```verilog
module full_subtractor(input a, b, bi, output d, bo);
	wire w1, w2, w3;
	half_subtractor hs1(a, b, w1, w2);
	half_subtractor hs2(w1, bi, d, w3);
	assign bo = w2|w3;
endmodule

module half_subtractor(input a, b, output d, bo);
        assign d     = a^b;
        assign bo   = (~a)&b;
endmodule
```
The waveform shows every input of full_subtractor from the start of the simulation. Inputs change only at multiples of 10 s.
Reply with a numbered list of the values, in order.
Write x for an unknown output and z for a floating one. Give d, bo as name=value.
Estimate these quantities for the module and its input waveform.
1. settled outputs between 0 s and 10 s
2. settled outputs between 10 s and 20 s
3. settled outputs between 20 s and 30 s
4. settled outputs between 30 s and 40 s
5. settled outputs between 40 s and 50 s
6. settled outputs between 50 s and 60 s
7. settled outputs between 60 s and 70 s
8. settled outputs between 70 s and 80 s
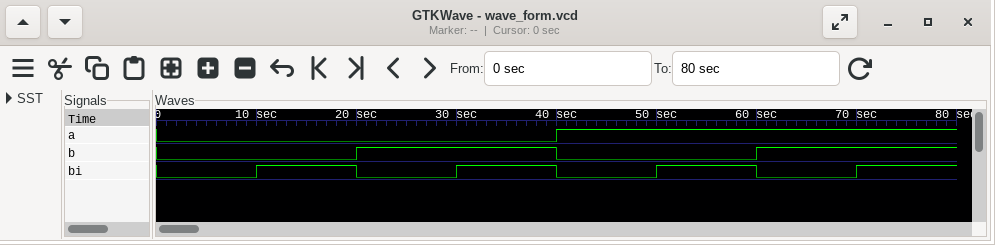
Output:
1. d=0, bo=0
2. d=1, bo=1
3. d=1, bo=1
4. d=0, bo=1
5. d=1, bo=0
6. d=0, bo=0
7. d=0, bo=0
8. d=1, bo=1
